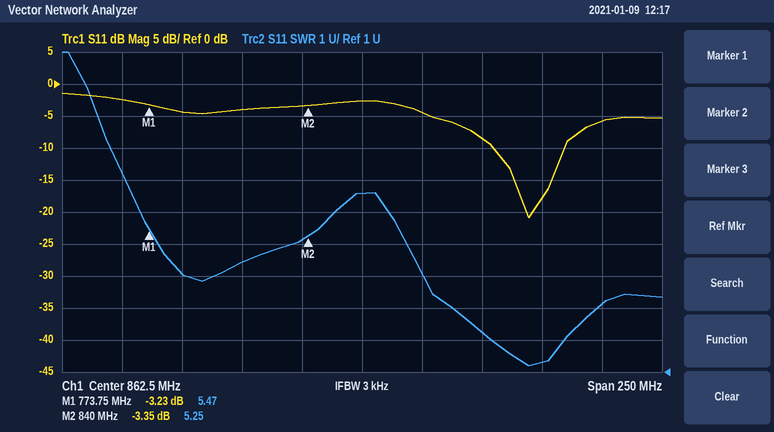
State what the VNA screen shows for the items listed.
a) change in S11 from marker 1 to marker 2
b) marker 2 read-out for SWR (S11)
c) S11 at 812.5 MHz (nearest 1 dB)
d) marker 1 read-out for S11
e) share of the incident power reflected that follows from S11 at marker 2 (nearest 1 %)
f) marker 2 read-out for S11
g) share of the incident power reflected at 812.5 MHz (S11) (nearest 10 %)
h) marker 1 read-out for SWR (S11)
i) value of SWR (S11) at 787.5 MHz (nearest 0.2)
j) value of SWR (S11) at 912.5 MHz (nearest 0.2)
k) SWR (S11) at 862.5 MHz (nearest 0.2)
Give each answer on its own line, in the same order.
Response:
-0.12 dB
5.25
-4 dB
-3.23 dB
46 %
-3.35 dB
40 %
5.47
4.0
2.2
6.6
